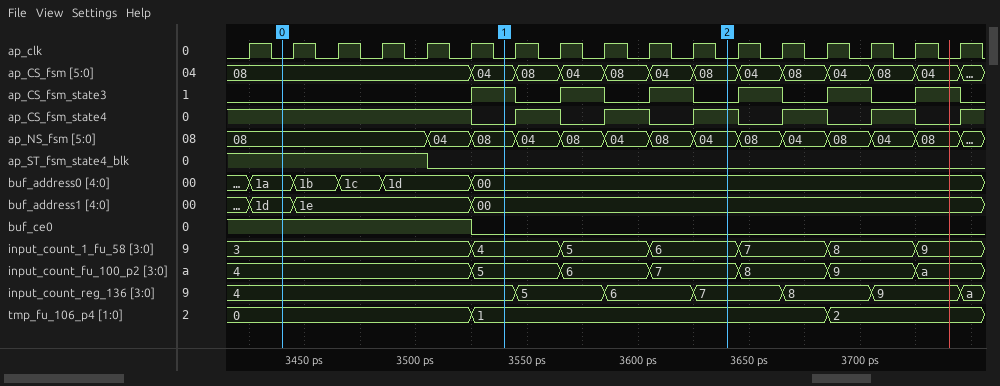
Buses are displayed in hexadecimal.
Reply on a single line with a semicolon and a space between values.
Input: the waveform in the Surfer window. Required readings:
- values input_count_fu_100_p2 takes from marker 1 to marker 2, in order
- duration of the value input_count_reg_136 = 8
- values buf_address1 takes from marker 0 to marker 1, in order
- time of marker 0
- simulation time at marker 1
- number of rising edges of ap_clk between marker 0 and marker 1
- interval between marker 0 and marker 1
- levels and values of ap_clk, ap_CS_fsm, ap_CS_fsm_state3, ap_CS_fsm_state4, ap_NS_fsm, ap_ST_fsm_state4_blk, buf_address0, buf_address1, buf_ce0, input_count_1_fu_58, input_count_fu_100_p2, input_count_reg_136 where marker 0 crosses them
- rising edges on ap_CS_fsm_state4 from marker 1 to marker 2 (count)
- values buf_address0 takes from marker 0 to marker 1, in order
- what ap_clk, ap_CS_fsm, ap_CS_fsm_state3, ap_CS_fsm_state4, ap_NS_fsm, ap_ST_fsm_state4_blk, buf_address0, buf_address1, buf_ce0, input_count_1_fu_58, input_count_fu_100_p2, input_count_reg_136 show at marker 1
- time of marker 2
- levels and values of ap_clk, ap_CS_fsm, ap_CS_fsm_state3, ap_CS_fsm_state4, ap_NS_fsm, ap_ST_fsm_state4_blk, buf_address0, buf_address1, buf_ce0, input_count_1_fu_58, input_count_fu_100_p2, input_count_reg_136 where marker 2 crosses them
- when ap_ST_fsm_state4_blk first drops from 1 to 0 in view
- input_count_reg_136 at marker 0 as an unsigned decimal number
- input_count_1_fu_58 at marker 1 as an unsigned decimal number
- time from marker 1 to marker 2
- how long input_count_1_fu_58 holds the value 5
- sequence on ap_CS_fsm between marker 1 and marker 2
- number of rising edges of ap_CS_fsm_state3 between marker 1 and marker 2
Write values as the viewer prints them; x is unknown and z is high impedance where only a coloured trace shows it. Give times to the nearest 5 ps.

5, 6, 7; 40 ps; 1d, 1e, 00; 3440 ps; 3540 ps; 5; 100 ps; ap_clk=0, ap_CS_fsm=08, ap_CS_fsm_state3=0, ap_CS_fsm_state4=1, ap_NS_fsm=08, ap_ST_fsm_state4_blk=1, buf_address0=1a, buf_address1=1d, buf_ce0=1, input_count_1_fu_58=3, input_count_fu_100_p2=4, input_count_reg_136=4; 3; 1a, 1b, 1c, 1d, 00; ap_clk=0, ap_CS_fsm=04, ap_CS_fsm_state3=1, ap_CS_fsm_state4=0, ap_NS_fsm=08, ap_ST_fsm_state4_blk=0, buf_address0=00, buf_address1=00, buf_ce0=0, input_count_1_fu_58=4, input_count_fu_100_p2=5, input_count_reg_136=4; 3640 ps; ap_clk=0, ap_CS_fsm=08, ap_CS_fsm_state3=0, ap_CS_fsm_state4=1, ap_NS_fsm=04, ap_ST_fsm_state4_blk=0, buf_address0=00, buf_address1=00, buf_ce0=0, input_count_1_fu_58=6, input_count_fu_100_p2=7, input_count_reg_136=7; 3505 ps; 4; 4; 100 ps; 40 ps; 04, 08, 04, 08, 04, 08; 2
